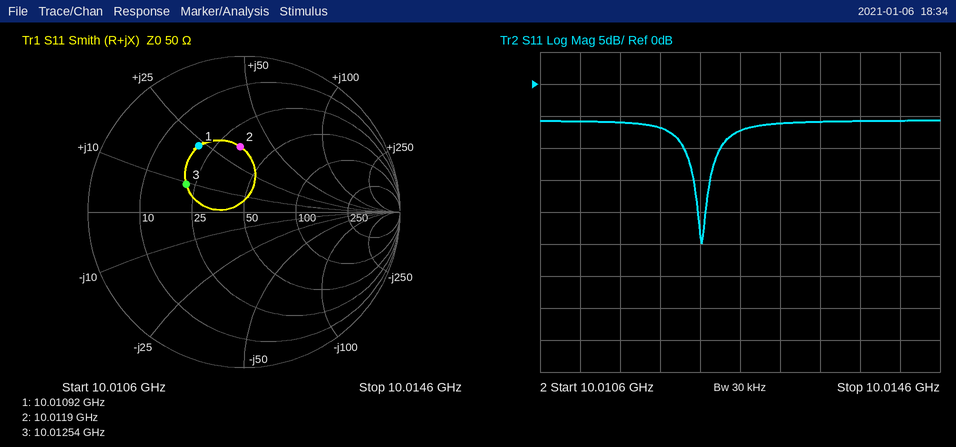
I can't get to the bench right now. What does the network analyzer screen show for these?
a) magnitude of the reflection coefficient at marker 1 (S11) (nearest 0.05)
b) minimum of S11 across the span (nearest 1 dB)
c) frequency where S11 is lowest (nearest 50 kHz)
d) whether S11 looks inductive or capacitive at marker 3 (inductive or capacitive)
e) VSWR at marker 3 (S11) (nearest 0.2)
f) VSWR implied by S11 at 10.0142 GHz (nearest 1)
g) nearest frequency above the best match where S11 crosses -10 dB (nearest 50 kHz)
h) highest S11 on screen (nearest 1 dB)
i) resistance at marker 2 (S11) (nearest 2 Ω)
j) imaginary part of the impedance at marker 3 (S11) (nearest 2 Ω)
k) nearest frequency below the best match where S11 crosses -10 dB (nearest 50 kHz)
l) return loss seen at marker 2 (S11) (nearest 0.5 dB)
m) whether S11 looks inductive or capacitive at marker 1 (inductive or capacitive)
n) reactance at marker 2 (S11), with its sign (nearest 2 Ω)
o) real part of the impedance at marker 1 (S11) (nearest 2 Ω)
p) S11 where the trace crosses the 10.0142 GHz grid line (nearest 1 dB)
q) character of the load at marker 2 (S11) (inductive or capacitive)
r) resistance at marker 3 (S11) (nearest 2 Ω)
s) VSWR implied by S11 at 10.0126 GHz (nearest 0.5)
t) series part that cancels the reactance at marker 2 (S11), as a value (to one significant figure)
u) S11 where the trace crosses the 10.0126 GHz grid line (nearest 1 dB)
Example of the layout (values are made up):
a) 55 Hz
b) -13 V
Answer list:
a) 0.50
b) -25 dB
c) 10.01220 GHz
d) inductive
e) 2.4
f) 3
g) 10.01240 GHz
h) -6 dB
i) 34 Ω
j) +10 Ω
k) 10.01205 GHz
l) 7.5 dB
m) inductive
n) +34 Ω
o) 20 Ω
p) -6 dB
q) inductive
r) 22 Ω
s) 2.5
t) 500 fF
u) -7 dB
